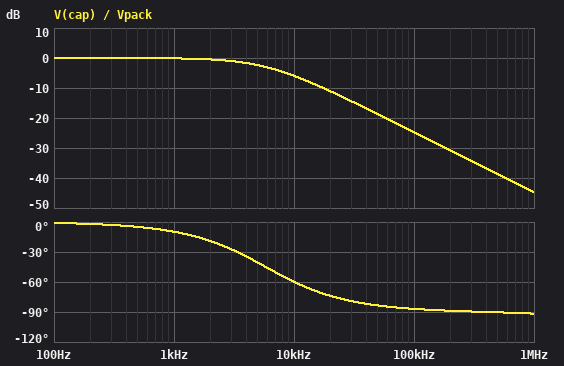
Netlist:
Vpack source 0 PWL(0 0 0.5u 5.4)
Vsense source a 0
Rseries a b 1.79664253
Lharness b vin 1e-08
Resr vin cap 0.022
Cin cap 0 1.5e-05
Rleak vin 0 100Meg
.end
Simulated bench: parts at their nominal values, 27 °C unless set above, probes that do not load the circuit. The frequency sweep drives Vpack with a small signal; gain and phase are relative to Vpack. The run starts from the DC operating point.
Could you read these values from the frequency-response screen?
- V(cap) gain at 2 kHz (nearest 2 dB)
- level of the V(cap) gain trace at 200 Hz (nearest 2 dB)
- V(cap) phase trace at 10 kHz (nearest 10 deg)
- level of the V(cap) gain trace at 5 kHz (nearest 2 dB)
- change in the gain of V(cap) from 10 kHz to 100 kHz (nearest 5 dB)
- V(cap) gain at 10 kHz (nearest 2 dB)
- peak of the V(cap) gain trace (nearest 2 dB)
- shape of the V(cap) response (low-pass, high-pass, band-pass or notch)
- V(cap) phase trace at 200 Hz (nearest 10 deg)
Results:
0 dB
0 dB
-60 deg
-2 dB
-20 dB
-6 dB
0 dB
low-pass
0 deg
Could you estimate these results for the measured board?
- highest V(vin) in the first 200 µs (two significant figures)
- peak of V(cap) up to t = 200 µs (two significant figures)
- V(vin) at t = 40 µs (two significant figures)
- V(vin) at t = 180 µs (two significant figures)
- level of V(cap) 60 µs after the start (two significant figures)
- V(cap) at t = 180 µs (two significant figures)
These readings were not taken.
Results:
5.4 V
5.4 V
4.2 V
5.4 V
4.8 V
5.4 V
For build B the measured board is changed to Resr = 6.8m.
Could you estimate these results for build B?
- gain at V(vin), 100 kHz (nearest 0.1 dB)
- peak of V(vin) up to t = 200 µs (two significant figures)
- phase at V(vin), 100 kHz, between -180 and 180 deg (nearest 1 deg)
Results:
-24.6 dB
5.4 V
-83 deg
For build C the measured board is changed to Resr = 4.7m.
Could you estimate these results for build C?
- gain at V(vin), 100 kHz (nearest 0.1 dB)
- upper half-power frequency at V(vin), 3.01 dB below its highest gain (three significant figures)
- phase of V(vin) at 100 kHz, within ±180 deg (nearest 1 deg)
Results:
-24.6 dB
5.89 kHz
-84 deg
